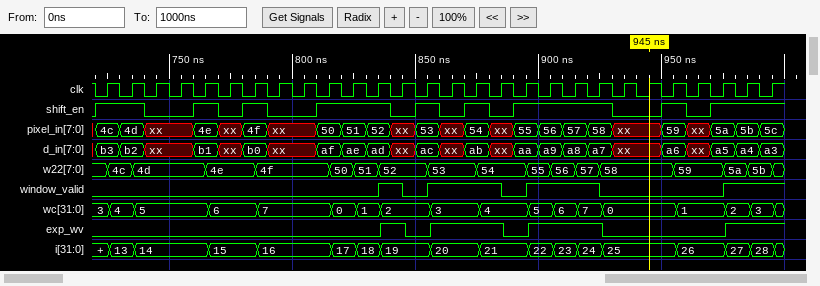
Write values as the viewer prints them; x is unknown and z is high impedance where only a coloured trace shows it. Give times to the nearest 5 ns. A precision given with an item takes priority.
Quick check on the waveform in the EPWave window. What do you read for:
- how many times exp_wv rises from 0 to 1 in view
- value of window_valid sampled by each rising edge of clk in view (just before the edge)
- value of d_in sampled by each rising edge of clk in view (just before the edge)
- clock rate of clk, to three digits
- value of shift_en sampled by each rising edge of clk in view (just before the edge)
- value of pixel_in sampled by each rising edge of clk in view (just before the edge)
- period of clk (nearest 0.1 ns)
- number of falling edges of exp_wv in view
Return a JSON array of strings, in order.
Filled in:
["4", "0 0 0 0 0 0 0 0 0 0 0 0 1 0 1 1 1 0 1 1 1 0 0 0 0 0 1 1", "b3, b2, xx, xx, b1, xx, b0, xx, xx, af, ae, ad, xx, ac, xx, ab, xx, aa, a9, a8, a7, xx, xx, a6, xx, a5, a4, a3", "100 MHz", "1 1 0 0 1 0 1 0 0 1 1 1 0 1 0 1 0 1 1 1 1 0 0 1 0 1 1 1", "4c, 4d, xx, xx, 4e, xx, 4f, xx, xx, 50, 51, 52, xx, 53, xx, 54, xx, 55, 56, 57, 58, xx, xx, 59, xx, 5a, 5b, 5c", "10 ns", "3"]
